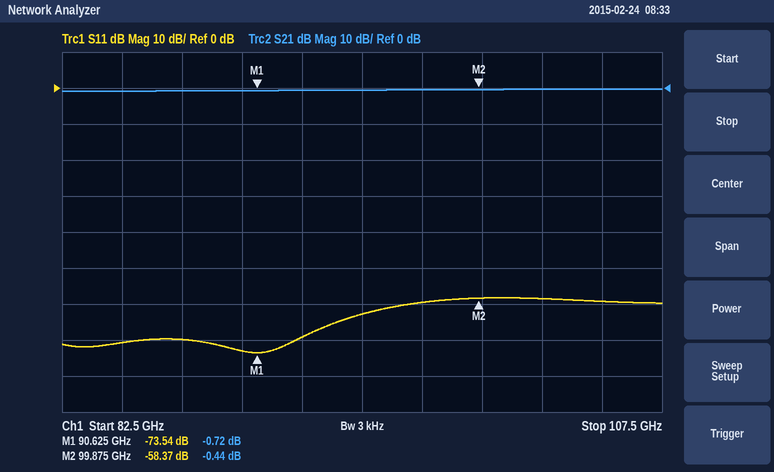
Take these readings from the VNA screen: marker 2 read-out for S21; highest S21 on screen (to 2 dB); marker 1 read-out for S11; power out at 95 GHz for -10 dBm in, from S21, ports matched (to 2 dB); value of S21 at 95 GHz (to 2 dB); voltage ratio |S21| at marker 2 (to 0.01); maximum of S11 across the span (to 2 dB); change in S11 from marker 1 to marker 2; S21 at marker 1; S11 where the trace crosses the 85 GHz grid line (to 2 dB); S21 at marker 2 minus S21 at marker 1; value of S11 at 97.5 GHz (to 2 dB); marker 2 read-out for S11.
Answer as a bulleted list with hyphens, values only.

- -0.44 dB
- 0 dB
- -73.54 dB
- -10 dBm
- 0 dB
- 0.95
- -58 dB
- 15.17 dB
- -0.72 dB
- -70 dB
- 0.28 dB
- -60 dB
- -58.37 dB
